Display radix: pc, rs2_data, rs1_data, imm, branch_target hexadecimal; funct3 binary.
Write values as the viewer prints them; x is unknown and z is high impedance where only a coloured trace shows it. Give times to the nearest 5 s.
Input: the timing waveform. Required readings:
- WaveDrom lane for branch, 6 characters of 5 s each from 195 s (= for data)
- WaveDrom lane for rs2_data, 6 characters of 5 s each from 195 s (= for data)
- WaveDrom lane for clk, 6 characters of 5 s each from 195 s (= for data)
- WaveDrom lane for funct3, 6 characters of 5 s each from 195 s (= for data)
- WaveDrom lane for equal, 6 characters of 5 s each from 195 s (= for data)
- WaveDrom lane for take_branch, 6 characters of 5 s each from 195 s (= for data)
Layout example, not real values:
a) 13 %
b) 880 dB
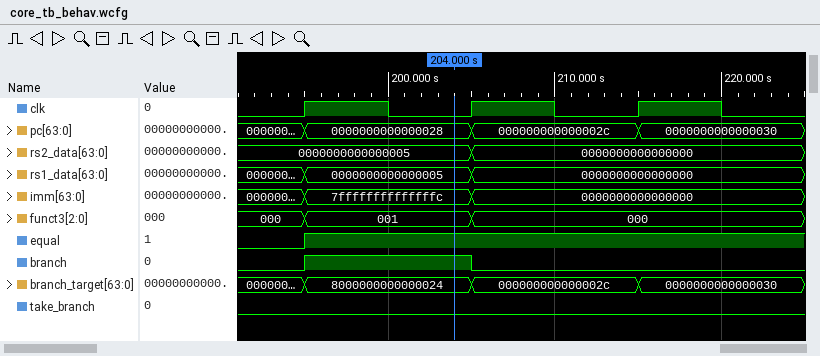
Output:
a) {name: 'branch', wave: '1.0...'}
b) {name: 'rs2_data', wave: '=.=...', data: '0000000000000005 0000000000000000'}
c) {name: 'clk', wave: '101010'}
d) {name: 'funct3', wave: '=.=...', data: '001 000'}
e) {name: 'equal', wave: '1.....'}
f) {name: 'take_branch', wave: '0.....'}
